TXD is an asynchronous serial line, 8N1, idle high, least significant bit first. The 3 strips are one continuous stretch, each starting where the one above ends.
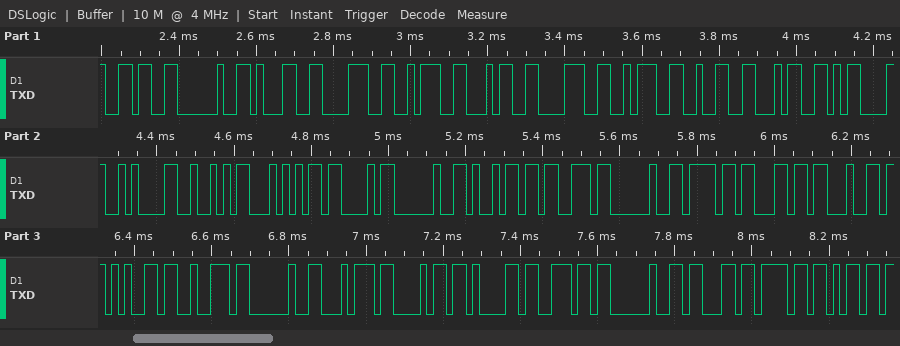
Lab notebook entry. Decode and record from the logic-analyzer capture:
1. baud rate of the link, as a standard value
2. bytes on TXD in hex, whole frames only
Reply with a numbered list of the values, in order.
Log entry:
1. 57600 baud
2. 36 20 31 38 3A 34 38 3A 32 34 0D 0A 52 54 43 20 69 73 20 6F 6C 64 65 72 20 74 68 61 6E 20 63 6F 6D
